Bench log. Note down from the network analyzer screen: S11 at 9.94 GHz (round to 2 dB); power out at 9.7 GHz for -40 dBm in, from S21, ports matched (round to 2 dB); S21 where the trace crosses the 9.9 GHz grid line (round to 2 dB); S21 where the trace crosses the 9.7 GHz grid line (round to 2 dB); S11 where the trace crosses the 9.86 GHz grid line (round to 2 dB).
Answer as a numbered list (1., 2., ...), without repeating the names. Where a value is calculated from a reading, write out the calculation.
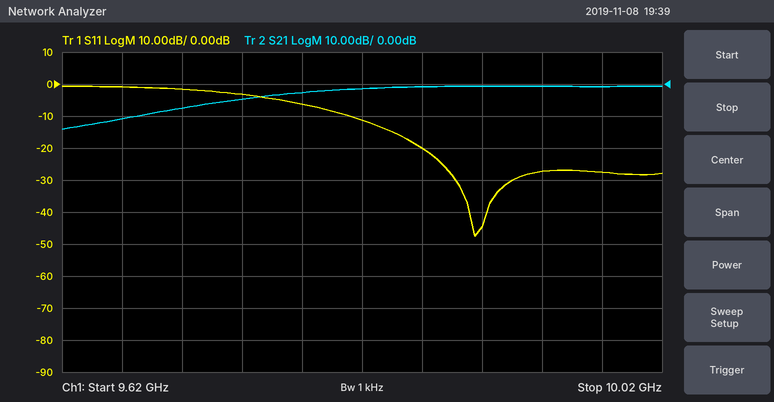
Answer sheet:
1. -28 dB
2. -40 dBm + (-8 dB) = -48 dBm
3. 0 dB
4. -8 dB
5. -20 dB
